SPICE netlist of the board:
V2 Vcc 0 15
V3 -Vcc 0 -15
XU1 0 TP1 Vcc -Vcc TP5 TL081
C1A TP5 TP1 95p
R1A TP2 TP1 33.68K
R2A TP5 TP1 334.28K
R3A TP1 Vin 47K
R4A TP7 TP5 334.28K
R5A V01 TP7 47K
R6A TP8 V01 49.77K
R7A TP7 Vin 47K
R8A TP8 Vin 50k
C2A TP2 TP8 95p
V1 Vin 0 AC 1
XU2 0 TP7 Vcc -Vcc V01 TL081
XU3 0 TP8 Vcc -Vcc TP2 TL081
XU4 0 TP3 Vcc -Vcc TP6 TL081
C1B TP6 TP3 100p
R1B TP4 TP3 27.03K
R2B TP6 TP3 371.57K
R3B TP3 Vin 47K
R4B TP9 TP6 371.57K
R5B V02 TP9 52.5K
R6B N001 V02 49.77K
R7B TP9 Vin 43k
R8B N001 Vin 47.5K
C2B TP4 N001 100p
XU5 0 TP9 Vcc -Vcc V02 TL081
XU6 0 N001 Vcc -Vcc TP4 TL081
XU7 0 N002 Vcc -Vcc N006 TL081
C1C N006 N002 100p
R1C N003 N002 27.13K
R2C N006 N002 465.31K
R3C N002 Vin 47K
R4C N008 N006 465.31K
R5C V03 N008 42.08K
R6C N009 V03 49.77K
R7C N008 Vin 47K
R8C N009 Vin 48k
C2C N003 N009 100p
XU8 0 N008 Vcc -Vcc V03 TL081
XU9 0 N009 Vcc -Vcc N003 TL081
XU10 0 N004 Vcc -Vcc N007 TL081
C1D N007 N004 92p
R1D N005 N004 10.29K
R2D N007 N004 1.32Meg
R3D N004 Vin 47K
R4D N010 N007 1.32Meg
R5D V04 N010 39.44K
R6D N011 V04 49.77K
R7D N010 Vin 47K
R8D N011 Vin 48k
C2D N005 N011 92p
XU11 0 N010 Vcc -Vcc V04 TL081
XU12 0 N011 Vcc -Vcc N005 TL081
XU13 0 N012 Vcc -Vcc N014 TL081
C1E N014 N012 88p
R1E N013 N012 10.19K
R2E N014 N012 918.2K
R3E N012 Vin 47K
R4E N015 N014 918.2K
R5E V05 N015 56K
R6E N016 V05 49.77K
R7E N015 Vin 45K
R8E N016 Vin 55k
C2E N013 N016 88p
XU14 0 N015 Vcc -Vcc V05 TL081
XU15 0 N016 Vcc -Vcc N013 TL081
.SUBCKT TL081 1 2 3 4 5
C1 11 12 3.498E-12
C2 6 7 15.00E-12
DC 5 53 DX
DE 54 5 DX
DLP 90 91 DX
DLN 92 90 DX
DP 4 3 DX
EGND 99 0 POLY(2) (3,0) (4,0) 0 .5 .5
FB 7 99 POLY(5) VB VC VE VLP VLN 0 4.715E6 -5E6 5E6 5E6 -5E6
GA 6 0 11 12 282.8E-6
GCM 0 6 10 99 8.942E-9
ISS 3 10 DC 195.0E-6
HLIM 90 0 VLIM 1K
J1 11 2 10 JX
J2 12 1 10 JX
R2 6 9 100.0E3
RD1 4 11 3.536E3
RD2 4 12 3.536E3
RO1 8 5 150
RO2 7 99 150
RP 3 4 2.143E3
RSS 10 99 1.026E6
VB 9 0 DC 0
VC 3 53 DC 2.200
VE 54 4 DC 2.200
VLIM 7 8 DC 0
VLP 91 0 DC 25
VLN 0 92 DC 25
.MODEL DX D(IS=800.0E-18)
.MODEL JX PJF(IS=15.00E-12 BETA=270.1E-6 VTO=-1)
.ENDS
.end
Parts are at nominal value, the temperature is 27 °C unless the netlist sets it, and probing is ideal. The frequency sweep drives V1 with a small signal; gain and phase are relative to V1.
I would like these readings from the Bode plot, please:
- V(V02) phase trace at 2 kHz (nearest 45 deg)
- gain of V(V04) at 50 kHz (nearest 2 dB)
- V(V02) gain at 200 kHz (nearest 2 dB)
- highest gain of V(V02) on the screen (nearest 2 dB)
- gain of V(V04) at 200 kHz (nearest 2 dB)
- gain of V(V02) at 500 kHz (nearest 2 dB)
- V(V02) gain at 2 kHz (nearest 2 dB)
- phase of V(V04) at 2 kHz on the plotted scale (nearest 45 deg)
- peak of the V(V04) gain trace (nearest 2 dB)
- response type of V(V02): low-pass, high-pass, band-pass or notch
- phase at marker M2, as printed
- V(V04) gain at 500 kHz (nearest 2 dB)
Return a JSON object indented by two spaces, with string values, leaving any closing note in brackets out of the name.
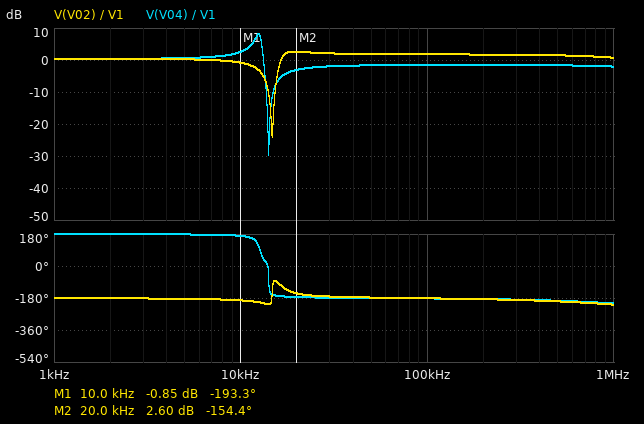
{
  "V(V02) phase trace at 2 kHz": "-180 deg",
  "gain of V(V04) at 50 kHz": "-2 dB",
  "V(V02) gain at 200 kHz": "2 dB",
  "highest gain of V(V02) on the screen": "2 dB",
  "gain of V(V04) at 200 kHz": "-2 dB",
  "gain of V(V02) at 500 kHz": "2 dB",
  "V(V02) gain at 2 kHz": "0 dB",
  "phase of V(V04) at 2 kHz on the plotted scale": "180 deg",
  "peak of the V(V04) gain trace": "8 dB",
  "response type of V(V02): low-pass, high-pass, band-pass or notch": "notch",
  "phase at marker M2, as printed": "-154.4 deg",
  "V(V04) gain at 500 kHz": "-2 dB"
}
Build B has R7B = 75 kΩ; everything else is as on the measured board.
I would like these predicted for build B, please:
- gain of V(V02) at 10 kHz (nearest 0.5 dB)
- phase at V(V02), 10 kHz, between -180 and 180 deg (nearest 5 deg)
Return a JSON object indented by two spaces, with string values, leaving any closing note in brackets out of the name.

{
  "gain of V(V02) at 10 kHz": "2.0 dB",
  "phase at V(V02), 10 kHz, between -180 and 180 deg": "160 deg"
}
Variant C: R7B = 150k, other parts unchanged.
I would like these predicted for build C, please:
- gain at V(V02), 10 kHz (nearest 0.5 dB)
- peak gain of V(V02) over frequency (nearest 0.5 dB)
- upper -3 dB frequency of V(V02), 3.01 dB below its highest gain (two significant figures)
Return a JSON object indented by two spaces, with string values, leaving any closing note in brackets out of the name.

{
  "gain at V(V02), 10 kHz": "3.5 dB",
  "peak gain of V(V02) over frequency": "9.5 dB",
  "upper -3 dB frequency of V(V02), 3.01 dB below its highest gain": "17 kHz"
}
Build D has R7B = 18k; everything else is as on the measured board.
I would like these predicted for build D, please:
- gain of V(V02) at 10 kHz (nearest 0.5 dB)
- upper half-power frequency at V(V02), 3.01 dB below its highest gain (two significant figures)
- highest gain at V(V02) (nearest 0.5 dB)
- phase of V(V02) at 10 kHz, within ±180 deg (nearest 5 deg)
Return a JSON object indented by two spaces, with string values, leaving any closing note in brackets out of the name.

{
  "gain of V(V02) at 10 kHz": "-6.0 dB",
  "upper half-power frequency at V(V02), 3.01 dB below its highest gain": "19 kHz",
  "highest gain at V(V02)": "18.5 dB",
  "phase of V(V02) at 10 kHz, within ±180 deg": "-85 deg"
}
